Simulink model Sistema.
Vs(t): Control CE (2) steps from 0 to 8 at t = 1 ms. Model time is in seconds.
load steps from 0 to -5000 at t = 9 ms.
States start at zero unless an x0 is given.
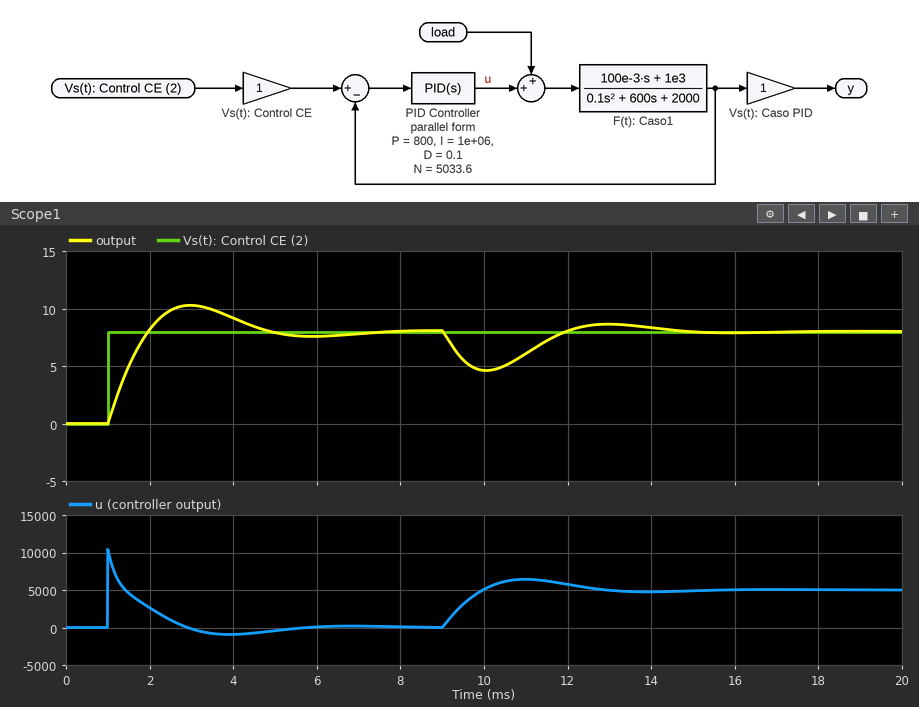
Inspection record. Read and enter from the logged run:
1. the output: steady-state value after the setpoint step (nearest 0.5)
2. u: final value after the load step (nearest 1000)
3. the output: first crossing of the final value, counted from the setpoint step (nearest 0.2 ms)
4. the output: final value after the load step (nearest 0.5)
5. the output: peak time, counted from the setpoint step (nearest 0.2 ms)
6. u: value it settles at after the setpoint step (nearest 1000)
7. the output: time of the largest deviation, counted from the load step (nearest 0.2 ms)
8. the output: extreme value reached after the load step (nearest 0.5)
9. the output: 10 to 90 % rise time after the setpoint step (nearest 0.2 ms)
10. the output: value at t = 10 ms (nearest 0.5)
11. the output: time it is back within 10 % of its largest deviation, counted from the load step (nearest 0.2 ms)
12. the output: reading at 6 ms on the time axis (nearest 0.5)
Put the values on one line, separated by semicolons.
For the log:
8.0; 5000; 1.0 ms; 8.0; 2.0 ms; 0; 1.0 ms; 4.5; 0.8 ms; 4.5; 5.0 ms; 7.5
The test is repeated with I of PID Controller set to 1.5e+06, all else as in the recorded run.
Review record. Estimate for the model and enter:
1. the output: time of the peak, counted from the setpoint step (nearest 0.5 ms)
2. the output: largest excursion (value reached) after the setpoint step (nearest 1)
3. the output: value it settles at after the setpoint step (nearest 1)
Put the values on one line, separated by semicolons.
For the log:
1.5 ms; 11; 8
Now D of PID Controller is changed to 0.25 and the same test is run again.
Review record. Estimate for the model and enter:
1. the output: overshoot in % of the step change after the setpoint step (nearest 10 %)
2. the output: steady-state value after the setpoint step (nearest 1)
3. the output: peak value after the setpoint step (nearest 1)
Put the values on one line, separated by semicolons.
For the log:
20 %; 8; 10
